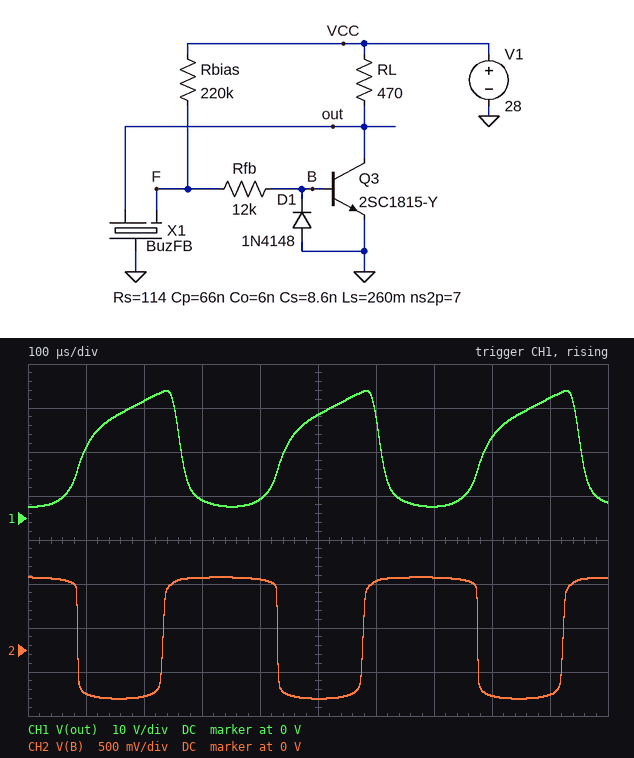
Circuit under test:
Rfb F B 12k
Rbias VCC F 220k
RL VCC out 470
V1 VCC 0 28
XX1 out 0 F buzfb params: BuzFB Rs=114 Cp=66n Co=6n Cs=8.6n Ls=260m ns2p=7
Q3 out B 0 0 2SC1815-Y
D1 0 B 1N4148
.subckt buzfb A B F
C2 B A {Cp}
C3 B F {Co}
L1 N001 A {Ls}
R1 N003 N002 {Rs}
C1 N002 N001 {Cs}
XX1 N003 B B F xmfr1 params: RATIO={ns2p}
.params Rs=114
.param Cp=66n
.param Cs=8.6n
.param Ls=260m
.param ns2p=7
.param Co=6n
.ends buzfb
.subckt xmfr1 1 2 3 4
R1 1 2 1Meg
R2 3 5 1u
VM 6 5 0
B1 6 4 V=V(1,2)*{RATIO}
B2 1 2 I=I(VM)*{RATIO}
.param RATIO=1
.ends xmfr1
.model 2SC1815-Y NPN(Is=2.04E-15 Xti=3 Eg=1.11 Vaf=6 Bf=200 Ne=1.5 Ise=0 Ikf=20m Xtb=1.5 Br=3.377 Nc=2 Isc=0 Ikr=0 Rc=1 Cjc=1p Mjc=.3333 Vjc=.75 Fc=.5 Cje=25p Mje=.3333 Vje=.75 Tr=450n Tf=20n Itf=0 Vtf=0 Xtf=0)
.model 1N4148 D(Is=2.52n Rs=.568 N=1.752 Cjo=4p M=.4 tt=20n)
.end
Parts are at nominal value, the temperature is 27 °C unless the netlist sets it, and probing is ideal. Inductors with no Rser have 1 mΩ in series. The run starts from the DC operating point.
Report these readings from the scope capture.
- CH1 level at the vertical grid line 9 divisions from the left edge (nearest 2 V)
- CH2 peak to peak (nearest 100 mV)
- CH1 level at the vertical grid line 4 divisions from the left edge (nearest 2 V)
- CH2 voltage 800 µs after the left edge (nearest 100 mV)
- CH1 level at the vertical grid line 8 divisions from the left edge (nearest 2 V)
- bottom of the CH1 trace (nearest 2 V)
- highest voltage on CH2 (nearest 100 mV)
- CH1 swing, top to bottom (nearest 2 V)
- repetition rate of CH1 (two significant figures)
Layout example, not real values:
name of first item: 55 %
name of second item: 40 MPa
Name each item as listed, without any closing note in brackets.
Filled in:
CH1 level at the vertical grid line 9 divisions from the left edge: 28 V
CH2 peak to peak: 1.4 V
CH1 level at the vertical grid line 4 divisions from the left edge: 4 V
CH2 voltage 800 µs after the left edge: -500 mV
CH1 level at the vertical grid line 8 divisions from the left edge: 18 V
bottom of the CH1 trace: 2 V
highest voltage on CH2: 800 mV
CH1 swing, top to bottom: 26 V
repetition rate of CH1: 2.9 kHz
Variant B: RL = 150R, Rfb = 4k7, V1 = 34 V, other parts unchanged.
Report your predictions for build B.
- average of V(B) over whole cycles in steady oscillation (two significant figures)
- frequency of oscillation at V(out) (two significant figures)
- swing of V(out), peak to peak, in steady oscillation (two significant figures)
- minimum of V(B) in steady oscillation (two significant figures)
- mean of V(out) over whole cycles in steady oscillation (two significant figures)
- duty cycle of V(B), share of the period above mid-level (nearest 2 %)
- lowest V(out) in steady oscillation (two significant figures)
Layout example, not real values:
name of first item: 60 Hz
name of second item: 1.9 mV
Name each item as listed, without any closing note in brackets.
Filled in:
average of V(B) over whole cycles in steady oscillation: 140 mV
frequency of oscillation at V(out): 3.3 kHz
swing of V(out), peak to peak, in steady oscillation: 32 V
minimum of V(B) in steady oscillation: -670 mV
mean of V(out) over whole cycles in steady oscillation: 18 V
duty cycle of V(B), share of the period above mid-level: 52 %
lowest V(out) in steady oscillation: 4.6 V
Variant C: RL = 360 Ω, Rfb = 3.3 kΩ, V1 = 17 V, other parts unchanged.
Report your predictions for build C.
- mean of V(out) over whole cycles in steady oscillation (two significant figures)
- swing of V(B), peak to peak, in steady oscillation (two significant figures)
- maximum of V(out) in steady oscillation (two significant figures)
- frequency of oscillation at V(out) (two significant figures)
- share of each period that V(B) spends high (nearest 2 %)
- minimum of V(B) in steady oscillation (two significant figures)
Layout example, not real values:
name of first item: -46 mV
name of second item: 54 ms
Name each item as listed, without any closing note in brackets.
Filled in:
mean of V(out) over whole cycles in steady oscillation: 6.1 V
swing of V(B), peak to peak, in steady oscillation: 1.5 V
maximum of V(out) in steady oscillation: 17 V
frequency of oscillation at V(out): 3.3 kHz
share of each period that V(B) spends high: 52 %
minimum of V(B) in steady oscillation: -630 mV
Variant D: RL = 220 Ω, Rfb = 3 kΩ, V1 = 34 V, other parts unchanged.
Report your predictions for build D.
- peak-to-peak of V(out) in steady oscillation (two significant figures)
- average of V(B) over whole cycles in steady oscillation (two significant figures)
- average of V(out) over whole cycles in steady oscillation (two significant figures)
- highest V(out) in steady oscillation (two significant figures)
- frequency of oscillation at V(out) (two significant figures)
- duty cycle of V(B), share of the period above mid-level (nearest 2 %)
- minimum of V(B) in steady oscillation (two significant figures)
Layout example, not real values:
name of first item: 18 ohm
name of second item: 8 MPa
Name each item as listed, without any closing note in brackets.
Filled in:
peak-to-peak of V(out) in steady oscillation: 33 V
average of V(B) over whole cycles in steady oscillation: 130 mV
average of V(out) over whole cycles in steady oscillation: 15 V
highest V(out) in steady oscillation: 35 V
frequency of oscillation at V(out): 3.3 kHz
duty cycle of V(B), share of the period above mid-level: 52 %
minimum of V(B) in steady oscillation: -680 mV
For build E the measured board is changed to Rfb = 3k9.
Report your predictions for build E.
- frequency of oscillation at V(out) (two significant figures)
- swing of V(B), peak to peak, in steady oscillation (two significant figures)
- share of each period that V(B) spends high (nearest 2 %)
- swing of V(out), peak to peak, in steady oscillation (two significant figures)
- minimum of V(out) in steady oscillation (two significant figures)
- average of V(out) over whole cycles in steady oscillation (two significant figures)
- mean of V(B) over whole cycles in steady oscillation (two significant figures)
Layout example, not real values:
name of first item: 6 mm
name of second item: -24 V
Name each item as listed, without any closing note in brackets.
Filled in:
frequency of oscillation at V(out): 3.3 kHz
swing of V(B), peak to peak, in steady oscillation: 1.5 V
share of each period that V(B) spends high: 52 %
swing of V(out), peak to peak, in steady oscillation: 27 V
minimum of V(out) in steady oscillation: 200 mV
average of V(out) over whole cycles in steady oscillation: 9.2 V
mean of V(B) over whole cycles in steady oscillation: 140 mV
